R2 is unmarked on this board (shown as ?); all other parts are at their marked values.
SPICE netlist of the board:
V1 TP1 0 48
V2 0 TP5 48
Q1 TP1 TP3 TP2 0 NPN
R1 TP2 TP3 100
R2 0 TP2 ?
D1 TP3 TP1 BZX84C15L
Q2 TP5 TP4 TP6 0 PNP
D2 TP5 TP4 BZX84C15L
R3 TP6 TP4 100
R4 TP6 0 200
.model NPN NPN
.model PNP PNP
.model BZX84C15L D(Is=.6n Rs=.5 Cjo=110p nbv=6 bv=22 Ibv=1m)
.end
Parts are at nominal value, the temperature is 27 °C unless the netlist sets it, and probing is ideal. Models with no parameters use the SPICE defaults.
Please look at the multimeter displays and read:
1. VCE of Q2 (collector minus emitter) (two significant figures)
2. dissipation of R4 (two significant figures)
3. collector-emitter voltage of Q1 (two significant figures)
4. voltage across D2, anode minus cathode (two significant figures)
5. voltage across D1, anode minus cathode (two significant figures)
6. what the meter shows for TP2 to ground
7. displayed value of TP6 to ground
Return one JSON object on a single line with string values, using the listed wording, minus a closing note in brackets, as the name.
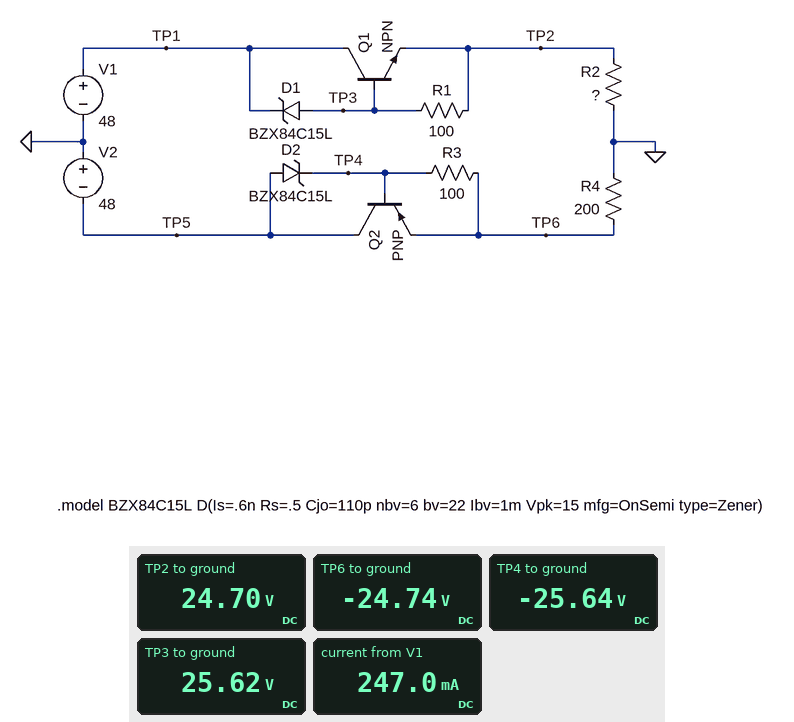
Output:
{"VCE of Q2 (collector minus emitter)": "-23 V", "dissipation of R4": "3.1 W", "collector-emitter voltage of Q1": "23 V", "voltage across D2, anode minus cathode": "-22 V", "voltage across D1, anode minus cathode": "-22 V", "what the meter shows for TP2 to ground": "24.70 V", "displayed value of TP6 to ground": "-24.74 V"}
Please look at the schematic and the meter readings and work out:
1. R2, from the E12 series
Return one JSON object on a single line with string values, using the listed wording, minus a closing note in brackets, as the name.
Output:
{"R2, from the E12 series": "100 Ω"}
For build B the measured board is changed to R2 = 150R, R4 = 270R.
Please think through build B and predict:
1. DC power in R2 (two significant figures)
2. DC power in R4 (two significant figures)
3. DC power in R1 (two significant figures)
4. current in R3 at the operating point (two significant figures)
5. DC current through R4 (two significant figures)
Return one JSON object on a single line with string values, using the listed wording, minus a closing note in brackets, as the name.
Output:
{"DC power in R2": "4.1 W", "DC power in R4": "2.3 W", "DC power in R1": "8.2 mW", "current in R3 at the operating point": "8.9 mA", "DC current through R4": "92 mA"}
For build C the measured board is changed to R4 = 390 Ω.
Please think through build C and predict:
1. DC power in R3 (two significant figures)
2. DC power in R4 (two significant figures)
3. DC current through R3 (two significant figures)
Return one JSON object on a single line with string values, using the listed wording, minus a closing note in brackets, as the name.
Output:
{"DC power in R3": "7.7 mW", "DC power in R4": "1.6 W", "DC current through R3": "8.8 mA"}
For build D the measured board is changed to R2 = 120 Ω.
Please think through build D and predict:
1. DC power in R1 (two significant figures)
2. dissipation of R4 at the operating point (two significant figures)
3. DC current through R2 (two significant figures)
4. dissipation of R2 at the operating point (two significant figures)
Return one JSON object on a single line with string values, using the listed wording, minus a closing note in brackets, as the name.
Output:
{"DC power in R1": "8.3 mW", "dissipation of R4 at the operating point": "3.1 W", "DC current through R2": "210 mA", "dissipation of R2 at the operating point": "5.1 W"}
